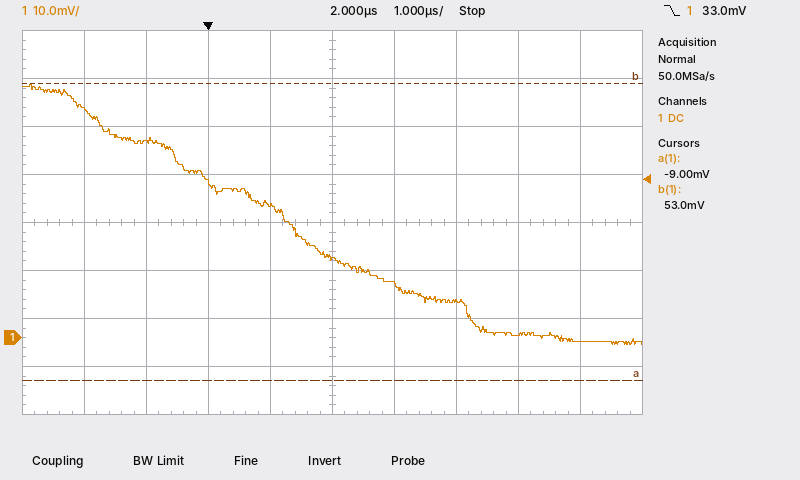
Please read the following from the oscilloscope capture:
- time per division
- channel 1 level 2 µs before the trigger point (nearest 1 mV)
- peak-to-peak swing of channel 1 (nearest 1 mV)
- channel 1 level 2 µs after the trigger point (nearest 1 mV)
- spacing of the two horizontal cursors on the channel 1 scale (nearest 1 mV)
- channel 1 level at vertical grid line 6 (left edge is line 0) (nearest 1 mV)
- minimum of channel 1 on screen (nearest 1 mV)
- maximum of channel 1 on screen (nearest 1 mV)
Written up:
1 µs
48 mV
54 mV
17 mV
62 mV
11 mV
-1 mV
53 mV
